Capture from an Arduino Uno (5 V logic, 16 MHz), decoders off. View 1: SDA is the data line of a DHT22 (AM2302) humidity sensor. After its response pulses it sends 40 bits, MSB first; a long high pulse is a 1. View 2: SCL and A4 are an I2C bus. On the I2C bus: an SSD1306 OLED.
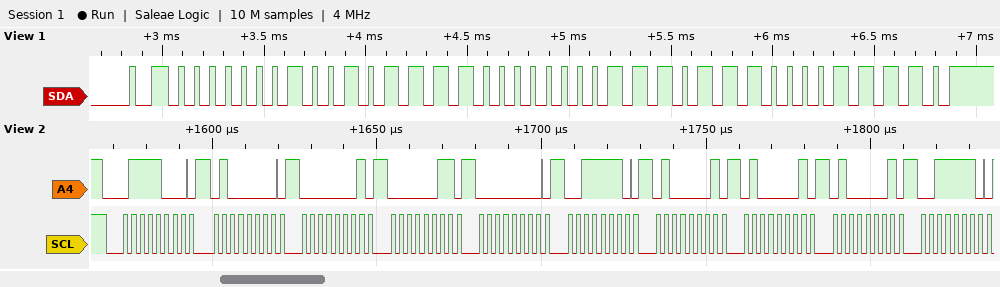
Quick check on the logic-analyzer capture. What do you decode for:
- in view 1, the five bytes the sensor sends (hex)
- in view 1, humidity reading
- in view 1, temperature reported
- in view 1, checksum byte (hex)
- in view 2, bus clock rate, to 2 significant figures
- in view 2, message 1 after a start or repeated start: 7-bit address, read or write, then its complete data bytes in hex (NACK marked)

01 2F 00 EE 1E
30.3 %
23.8 °C
0x1E
400 kHz
0x3C write: 40 01 03 00 3E 41 41 41 3E
